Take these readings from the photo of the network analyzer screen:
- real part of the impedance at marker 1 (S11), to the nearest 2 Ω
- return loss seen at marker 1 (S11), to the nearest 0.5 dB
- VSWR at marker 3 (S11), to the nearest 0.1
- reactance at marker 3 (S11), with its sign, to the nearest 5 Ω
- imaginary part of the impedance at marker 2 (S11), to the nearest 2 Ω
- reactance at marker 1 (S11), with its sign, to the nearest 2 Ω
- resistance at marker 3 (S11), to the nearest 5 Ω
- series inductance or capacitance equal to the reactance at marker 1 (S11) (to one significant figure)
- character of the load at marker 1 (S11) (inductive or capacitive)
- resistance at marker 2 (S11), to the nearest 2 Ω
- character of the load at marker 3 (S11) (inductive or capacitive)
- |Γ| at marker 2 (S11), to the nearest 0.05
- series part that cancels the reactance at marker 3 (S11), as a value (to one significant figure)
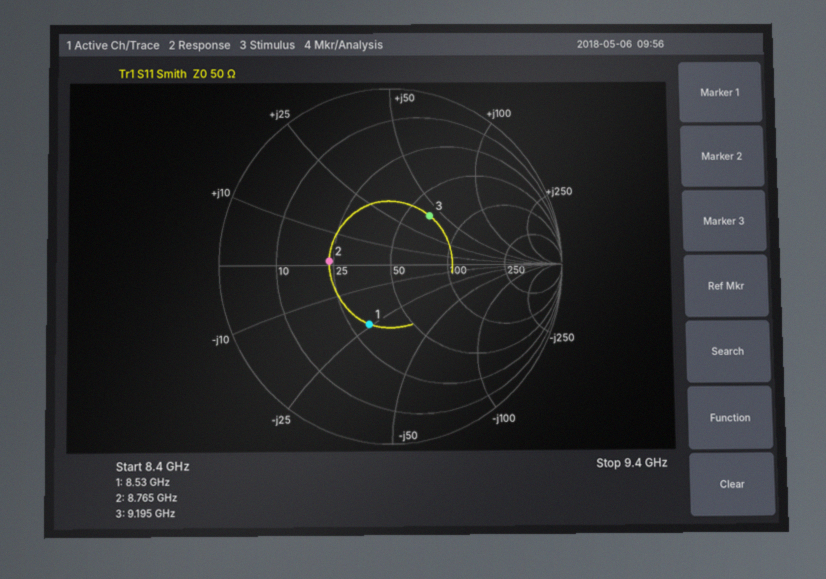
32 Ω
9.0 dB
2.1
+40 Ω
+2 Ω
-24 Ω
65 Ω
800 fF
capacitive
24 Ω
inductive
0.35
400 fF
